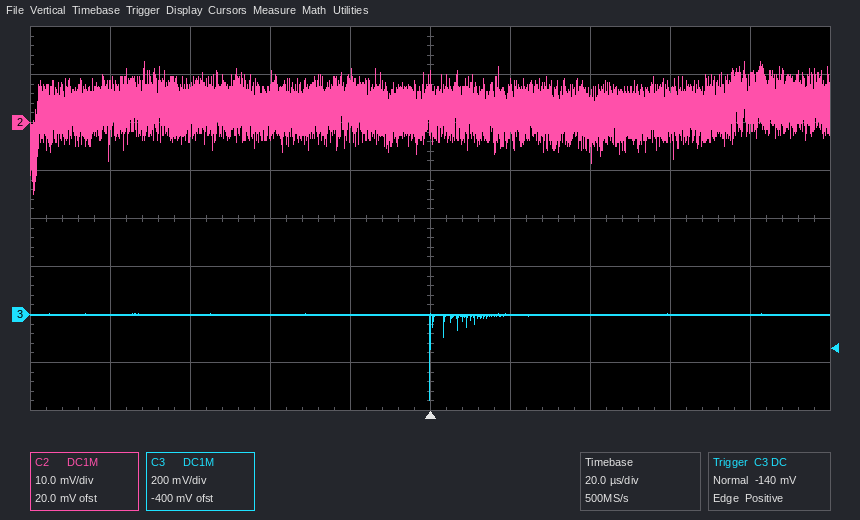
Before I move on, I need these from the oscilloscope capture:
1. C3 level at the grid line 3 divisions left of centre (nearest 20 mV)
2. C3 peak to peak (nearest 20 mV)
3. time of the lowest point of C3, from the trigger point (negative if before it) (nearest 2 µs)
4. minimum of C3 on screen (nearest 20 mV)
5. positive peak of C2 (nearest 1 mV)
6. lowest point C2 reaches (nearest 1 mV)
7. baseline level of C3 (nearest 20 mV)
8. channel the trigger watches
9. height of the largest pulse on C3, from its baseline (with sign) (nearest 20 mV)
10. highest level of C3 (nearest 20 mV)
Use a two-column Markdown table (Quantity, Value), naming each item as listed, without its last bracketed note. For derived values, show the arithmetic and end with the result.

| Quantity | Value |
|---|---|
| C3 level at the grid line 3 divisions left of centre | 0 mV |
| C3 peak to peak | 0 mV − (-360 mV) = 360 mV |
| time of the lowest point of C3, from the trigger point (negative if before it) | 0 µs |
| minimum of C3 on screen | -360 mV |
| positive peak of C2 | 13 mV |
| lowest point C2 reaches | -15 mV |
| baseline level of C3 | 0 mV |
| channel the trigger watches | C3 |
| height of the largest pulse on C3, from its baseline (with sign) | -360 mV − (0 mV) = -360 mV |
| highest level of C3 | 0 mV |
